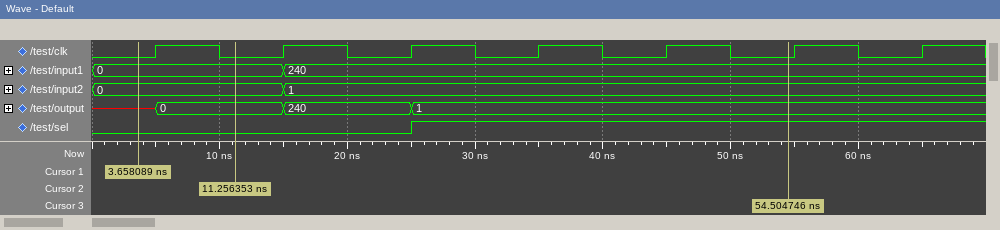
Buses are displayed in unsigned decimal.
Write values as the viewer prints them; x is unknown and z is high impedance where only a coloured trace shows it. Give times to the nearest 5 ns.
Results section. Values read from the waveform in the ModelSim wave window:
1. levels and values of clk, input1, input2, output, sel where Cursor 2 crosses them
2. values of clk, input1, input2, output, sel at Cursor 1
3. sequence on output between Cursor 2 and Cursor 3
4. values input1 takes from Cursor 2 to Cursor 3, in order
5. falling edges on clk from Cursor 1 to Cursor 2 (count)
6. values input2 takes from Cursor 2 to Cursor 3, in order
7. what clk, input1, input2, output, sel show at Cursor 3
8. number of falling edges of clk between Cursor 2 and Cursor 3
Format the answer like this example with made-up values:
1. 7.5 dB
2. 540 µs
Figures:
1. clk=0, input1=0, input2=0, output=0, sel=0
2. clk=0, input1=0, input2=0, output=x, sel=0
3. 0, 240, 1
4. 0, 240
5. 1
6. 0, 1
7. clk=0, input1=240, input2=1, output=1, sel=1
8. 4
